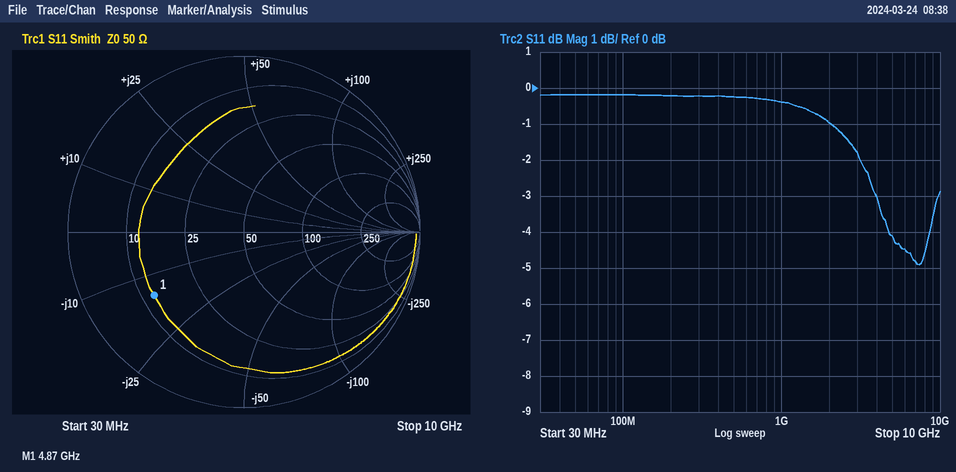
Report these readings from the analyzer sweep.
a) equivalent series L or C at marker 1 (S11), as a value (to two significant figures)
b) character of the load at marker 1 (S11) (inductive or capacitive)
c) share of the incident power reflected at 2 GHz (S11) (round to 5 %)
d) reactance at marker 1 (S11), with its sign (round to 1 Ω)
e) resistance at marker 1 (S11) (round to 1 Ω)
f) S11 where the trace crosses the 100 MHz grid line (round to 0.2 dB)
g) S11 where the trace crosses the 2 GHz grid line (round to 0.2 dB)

2.2 pF
capacitive
80 %
-15 Ω
13 Ω
-0.2 dB
-1.0 dB
